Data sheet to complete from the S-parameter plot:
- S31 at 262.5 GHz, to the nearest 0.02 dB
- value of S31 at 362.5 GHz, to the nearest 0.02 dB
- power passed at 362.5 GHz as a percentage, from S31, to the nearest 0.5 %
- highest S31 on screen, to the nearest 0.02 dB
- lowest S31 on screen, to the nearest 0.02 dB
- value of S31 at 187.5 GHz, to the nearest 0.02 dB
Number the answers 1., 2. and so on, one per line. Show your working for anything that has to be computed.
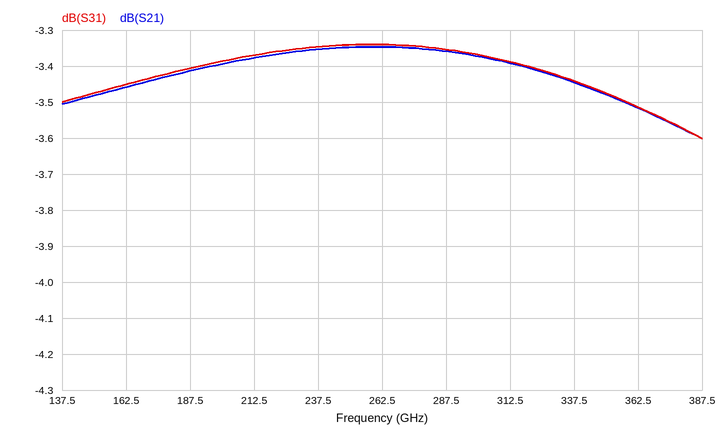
1. -3.34 dB
2. -3.52 dB
3. 10^(-3.52/10) ≈ 44.5 %
4. -3.34 dB
5. -3.60 dB
6. -3.40 dB
